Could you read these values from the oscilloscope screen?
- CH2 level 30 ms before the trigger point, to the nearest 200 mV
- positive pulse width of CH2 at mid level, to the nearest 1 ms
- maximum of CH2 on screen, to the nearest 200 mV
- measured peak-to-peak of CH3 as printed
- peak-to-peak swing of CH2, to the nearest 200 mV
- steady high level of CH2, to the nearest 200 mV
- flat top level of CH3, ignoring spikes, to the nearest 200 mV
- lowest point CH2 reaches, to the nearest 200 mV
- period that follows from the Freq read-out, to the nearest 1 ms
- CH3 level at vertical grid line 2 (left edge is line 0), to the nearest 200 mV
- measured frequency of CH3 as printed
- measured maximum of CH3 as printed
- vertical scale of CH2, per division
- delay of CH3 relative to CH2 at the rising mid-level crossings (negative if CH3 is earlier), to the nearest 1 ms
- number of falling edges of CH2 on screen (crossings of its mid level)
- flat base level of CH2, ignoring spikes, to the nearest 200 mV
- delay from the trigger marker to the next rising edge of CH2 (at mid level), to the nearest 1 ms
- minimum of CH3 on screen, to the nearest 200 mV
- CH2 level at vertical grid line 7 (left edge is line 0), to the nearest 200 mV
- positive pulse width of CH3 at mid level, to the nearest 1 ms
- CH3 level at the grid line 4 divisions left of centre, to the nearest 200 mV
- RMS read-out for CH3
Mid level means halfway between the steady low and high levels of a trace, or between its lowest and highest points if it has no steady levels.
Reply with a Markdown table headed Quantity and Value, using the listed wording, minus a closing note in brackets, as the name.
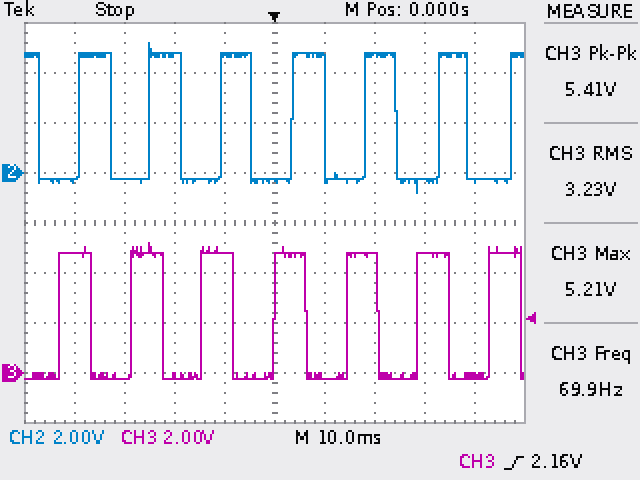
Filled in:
| Quantity | Value |
|---|---|
| CH2 level 30 ms before the trigger point, to the nearest 200 mV | -200 mV |
| positive pulse width of CH2 at mid level, to the nearest 1 ms | 6 ms |
| maximum of CH2 on screen, to the nearest 200 mV | 5.2 V |
| measured peak-to-peak of CH3 as printed | 5.41 V |
| peak-to-peak swing of CH2, to the nearest 200 mV | 6.0 V |
| steady high level of CH2, to the nearest 200 mV | 4.8 V |
| flat top level of CH3, ignoring spikes, to the nearest 200 mV | 4.8 V |
| lowest point CH2 reaches, to the nearest 200 mV | -800 mV |
| period that follows from the Freq read-out, to the nearest 1 ms | 14 ms |
| CH3 level at vertical grid line 2 (left edge is line 0), to the nearest 200 mV | -200 mV |
| measured frequency of CH3 as printed | 69.9 Hz |
| measured maximum of CH3 as printed | 5.21 V |
| vertical scale of CH2, per division | 2 V |
| delay of CH3 relative to CH2 at the rising mid-level crossings (negative if CH3 is earlier), to the nearest 1 ms | -4 ms |
| number of falling edges of CH2 on screen | 7 |
| flat base level of CH2, ignoring spikes, to the nearest 200 mV | -200 mV |
| delay from the trigger marker to the next rising edge of CH2 (at mid level), to the nearest 1 ms | 4 ms |
| minimum of CH3 on screen, to the nearest 200 mV | -200 mV |
| CH2 level at vertical grid line 7 (left edge is line 0), to the nearest 200 mV | 4.8 V |
| positive pulse width of CH3 at mid level, to the nearest 1 ms | 6 ms |
| CH3 level at the grid line 4 divisions left of centre, to the nearest 200 mV | 4.8 V |
| RMS read-out for CH3 | 3.23 V |
